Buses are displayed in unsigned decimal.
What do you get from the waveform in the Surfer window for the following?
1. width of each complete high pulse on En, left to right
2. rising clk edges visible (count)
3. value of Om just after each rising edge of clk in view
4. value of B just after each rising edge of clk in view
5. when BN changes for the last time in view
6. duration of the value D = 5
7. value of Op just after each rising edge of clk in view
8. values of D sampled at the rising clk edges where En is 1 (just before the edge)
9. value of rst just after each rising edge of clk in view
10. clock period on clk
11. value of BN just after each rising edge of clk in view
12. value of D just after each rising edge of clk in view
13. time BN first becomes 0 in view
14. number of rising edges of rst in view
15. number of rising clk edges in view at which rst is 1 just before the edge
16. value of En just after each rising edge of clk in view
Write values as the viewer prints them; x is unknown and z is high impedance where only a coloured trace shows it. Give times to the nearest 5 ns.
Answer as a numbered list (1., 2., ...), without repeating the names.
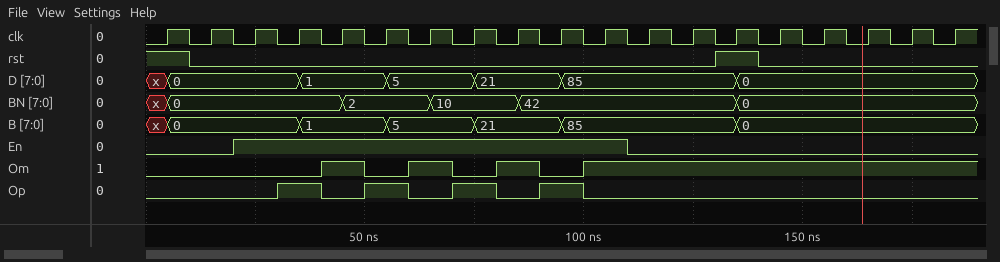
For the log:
1. 90 ns
2. 19
3. 0 0 0 0 1 0 1 0 1 0 1 1 1 1 1 1 1 1 1
4. 0, 0, 0, 1, 1, 5, 5, 21, 21, 85, 85, 85, 85, 0, 0, 0, 0, 0, 0
5. 135 ns
6. 20 ns
7. 0 0 0 1 0 1 0 1 0 1 0 0 0 0 0 0 0 0 0
8. 0, 0, 1, 1, 5, 5, 21, 21, 85
9. 1 0 0 0 0 0 0 0 0 0 0 0 0 1 0 0 0 0 0
10. 10 ns
11. 0, 0, 0, 0, 2, 2, 10, 10, 42, 42, 42, 42, 42, 0, 0, 0, 0, 0, 0
12. 0, 0, 0, 1, 1, 5, 5, 21, 21, 85, 85, 85, 85, 0, 0, 0, 0, 0, 0
13. 5 ns
14. 1
15. 2
16. 0 0 1 1 1 1 1 1 1 1 1 0 0 0 0 0 0 0 0
